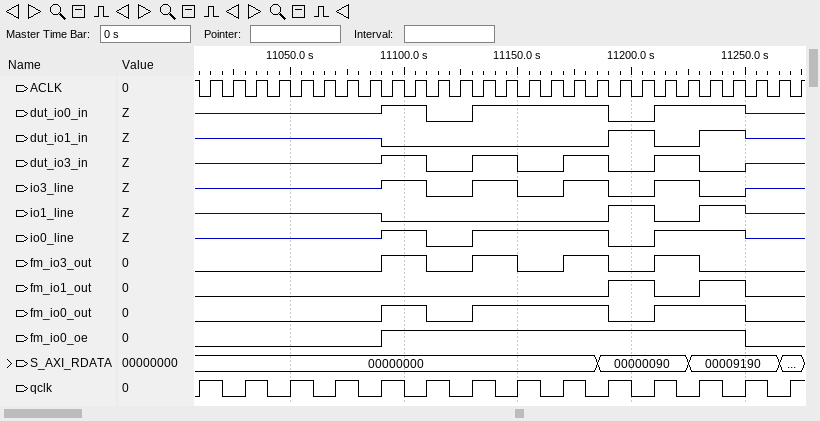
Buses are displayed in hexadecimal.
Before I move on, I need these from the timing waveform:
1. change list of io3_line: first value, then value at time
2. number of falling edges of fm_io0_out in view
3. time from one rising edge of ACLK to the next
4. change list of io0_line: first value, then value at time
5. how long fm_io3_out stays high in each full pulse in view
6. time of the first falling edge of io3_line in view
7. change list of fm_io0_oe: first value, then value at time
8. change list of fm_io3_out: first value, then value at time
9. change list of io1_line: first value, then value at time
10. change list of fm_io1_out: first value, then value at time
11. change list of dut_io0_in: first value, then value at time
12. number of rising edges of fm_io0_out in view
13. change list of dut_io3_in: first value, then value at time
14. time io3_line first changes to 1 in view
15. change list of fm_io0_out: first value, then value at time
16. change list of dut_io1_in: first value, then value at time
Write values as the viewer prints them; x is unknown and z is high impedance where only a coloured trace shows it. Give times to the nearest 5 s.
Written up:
z, 1 at 11090 s, 0 at 11110 s, 1 at 11130 s, 0 at 11150 s, 1 at 11170 s, 0 at 11190 s, 1 at 11210 s, 0 at 11230 s, z at 11250 s
3
10 s
z, 1 at 11090 s, 0 at 11110 s, 1 at 11130 s, 0 at 11190 s, 1 at 11210 s, z at 11250 s
20 s, 20 s, 20 s, 20 s
11110 s
0, 1 at 11090 s, 0 at 11250 s
0, 1 at 11090 s, 0 at 11110 s, 1 at 11130 s, 0 at 11150 s, 1 at 11170 s, 0 at 11190 s, 1 at 11210 s, 0 at 11230 s
z, 0 at 11090 s, 1 at 11190 s, 0 at 11210 s, 1 at 11230 s, z at 11250 s
0, 1 at 11190 s, 0 at 11210 s, 1 at 11230 s, 0 at 11250 s
z, 1 at 11090 s, 0 at 11110 s, 1 at 11130 s, 0 at 11190 s, 1 at 11210 s, z at 11250 s
3
z, 1 at 11090 s, 0 at 11110 s, 1 at 11130 s, 0 at 11150 s, 1 at 11170 s, 0 at 11190 s, 1 at 11210 s, 0 at 11230 s, z at 11250 s
11090 s
0, 1 at 11090 s, 0 at 11110 s, 1 at 11130 s, 0 at 11190 s, 1 at 11210 s, 0 at 11250 s
z, 0 at 11090 s, 1 at 11190 s, 0 at 11210 s, 1 at 11230 s, z at 11250 s
